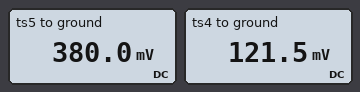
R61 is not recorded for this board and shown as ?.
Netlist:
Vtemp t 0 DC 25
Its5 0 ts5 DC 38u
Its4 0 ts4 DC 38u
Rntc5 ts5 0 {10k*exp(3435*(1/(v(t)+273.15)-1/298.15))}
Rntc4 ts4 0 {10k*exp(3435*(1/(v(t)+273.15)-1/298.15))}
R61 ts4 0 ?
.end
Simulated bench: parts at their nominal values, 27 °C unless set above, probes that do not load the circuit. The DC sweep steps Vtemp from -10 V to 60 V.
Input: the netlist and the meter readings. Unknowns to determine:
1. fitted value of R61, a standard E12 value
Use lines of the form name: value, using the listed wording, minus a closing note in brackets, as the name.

fitted value of R61, a standard E12 value: 4.7 kΩ
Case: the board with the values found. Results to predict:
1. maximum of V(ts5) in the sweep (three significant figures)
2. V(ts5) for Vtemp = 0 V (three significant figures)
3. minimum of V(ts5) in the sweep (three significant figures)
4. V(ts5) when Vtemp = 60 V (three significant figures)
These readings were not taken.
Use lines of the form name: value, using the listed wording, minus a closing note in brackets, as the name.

maximum of V(ts5) in the sweep: 1.76 V
V(ts5) for Vtemp = 0 V: 1.09 V
minimum of V(ts5) in the sweep: 113 mV
V(ts5) when Vtemp = 60 V: 113 mV
